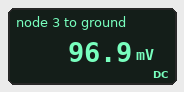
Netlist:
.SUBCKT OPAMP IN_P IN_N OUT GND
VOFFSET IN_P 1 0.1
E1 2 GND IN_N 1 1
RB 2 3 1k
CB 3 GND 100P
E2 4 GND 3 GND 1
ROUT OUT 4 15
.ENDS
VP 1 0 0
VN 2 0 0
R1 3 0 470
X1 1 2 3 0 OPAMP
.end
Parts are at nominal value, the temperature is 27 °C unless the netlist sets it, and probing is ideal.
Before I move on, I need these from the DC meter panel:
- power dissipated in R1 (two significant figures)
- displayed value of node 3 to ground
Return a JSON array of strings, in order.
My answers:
["20 µW", "96.9 mV"]
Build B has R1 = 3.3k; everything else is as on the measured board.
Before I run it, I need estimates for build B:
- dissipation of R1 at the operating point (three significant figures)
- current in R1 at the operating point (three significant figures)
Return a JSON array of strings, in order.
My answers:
["3.00 µW", "30.2 µA"]
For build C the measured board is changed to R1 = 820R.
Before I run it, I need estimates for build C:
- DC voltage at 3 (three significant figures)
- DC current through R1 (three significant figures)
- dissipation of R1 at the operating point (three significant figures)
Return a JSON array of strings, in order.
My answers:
["98.2 mV", "120 µA", "11.8 µW"]
